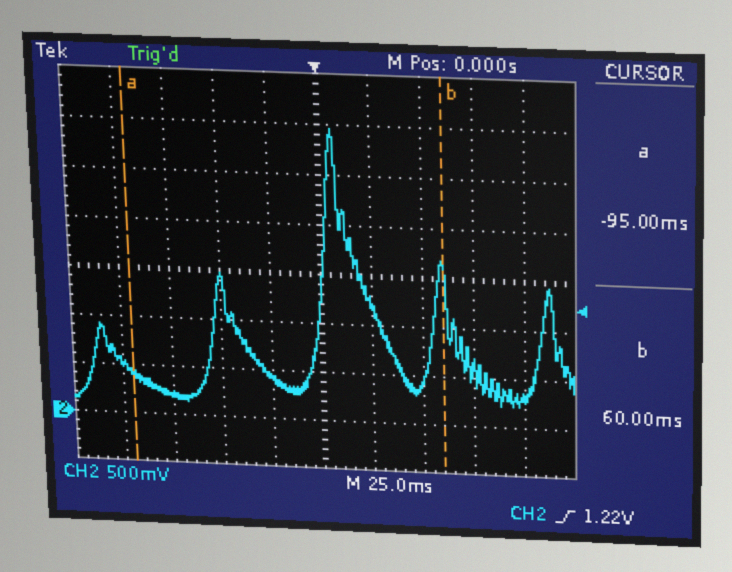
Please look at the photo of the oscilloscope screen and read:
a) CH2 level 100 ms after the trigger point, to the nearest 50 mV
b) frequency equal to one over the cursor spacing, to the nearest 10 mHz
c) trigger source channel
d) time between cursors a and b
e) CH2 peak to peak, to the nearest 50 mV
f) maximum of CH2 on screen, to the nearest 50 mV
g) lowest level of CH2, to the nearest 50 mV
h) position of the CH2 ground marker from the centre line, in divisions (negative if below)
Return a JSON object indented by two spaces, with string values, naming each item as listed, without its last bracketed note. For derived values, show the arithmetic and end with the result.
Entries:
{
  "CH2 level 100 ms after the trigger point, to the nearest 50 mV": "300 mV",
  "frequency equal to one over the cursor spacing, to the nearest 10 mHz": "1 / 155.0 ms ≈ 6.45 Hz",
  "trigger source channel": "CH2",
  "time between cursors a and b": "60 ms − (-95 ms) = 155.0 ms",
  "CH2 peak to peak, to the nearest 50 mV": "2.95 V − (150 mV) = 2.80 V",
  "maximum of CH2 on screen, to the nearest 50 mV": "2.95 V",
  "lowest level of CH2, to the nearest 50 mV": "150 mV",
  "position of the CH2 ground marker from the centre line, in divisions": "-3.0 div"
}
